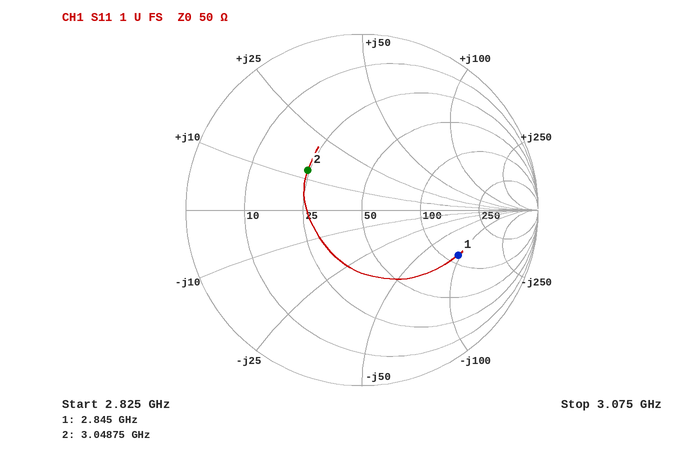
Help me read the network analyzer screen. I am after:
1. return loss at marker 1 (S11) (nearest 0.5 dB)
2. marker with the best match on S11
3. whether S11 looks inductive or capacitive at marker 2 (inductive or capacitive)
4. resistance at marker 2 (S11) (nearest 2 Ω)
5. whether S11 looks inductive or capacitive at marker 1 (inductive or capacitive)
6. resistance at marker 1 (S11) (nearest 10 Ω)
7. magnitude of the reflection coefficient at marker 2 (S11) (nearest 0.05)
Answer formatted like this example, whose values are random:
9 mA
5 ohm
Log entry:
4.5 dB
marker 2
inductive
24 Ω
capacitive
120 Ω
0.40
